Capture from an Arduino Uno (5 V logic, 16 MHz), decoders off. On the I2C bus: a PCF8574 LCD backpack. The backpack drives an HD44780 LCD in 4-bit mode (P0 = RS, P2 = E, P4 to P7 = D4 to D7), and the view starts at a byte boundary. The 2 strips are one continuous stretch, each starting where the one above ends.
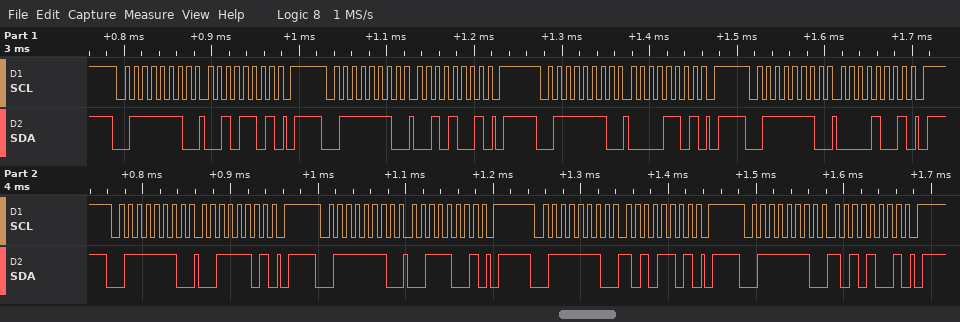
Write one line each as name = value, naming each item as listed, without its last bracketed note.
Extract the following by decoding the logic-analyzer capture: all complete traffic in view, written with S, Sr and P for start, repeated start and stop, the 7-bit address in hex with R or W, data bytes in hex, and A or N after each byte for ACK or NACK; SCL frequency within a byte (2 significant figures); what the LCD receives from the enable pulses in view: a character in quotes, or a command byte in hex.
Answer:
all complete traffic in view, written with S, Sr and P for start, repeated start and stop, the 7-bit address in hex with R or W, data bytes in hex, and A or N after each byte for ACK or NACK = S 3FW A 2D A P S 3FW A 29 A P S 3FW A 0D A P S 3FW A 09 A P S 3FW A 3D A P S 3FW A 39 A P S 3FW A AD A P S 3FW A A9 A P
SCL frequency within a byte = 100 kHz
what the LCD receives from the enable pulses in view: a character in quotes, or a command byte in hex = ' ' ':'
